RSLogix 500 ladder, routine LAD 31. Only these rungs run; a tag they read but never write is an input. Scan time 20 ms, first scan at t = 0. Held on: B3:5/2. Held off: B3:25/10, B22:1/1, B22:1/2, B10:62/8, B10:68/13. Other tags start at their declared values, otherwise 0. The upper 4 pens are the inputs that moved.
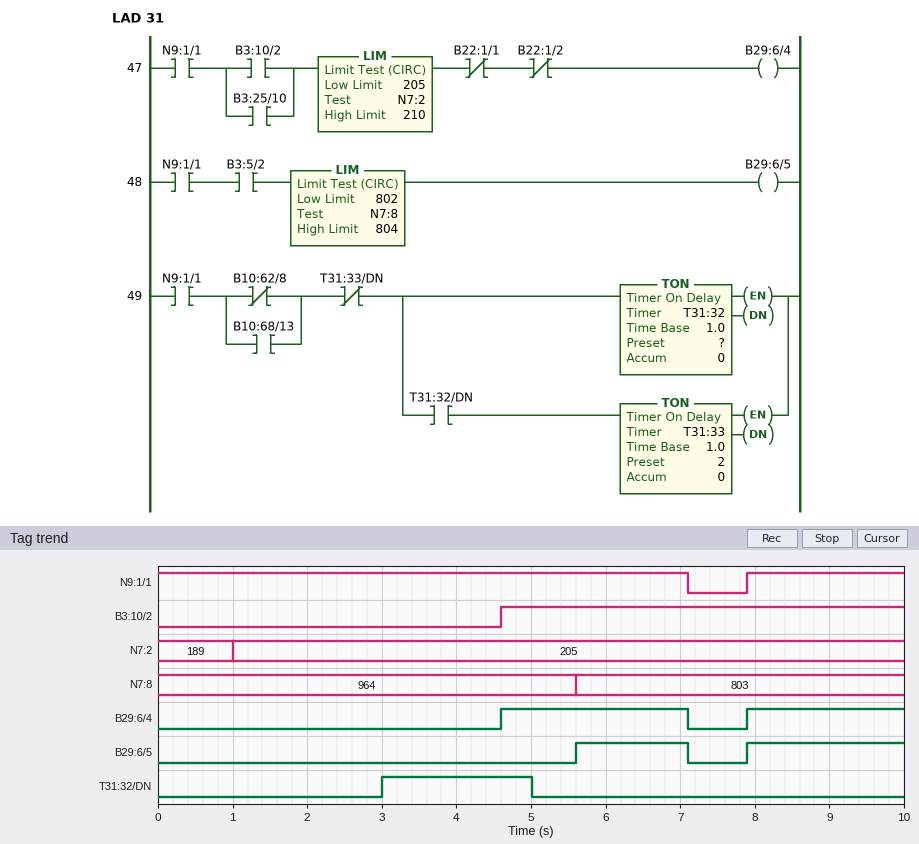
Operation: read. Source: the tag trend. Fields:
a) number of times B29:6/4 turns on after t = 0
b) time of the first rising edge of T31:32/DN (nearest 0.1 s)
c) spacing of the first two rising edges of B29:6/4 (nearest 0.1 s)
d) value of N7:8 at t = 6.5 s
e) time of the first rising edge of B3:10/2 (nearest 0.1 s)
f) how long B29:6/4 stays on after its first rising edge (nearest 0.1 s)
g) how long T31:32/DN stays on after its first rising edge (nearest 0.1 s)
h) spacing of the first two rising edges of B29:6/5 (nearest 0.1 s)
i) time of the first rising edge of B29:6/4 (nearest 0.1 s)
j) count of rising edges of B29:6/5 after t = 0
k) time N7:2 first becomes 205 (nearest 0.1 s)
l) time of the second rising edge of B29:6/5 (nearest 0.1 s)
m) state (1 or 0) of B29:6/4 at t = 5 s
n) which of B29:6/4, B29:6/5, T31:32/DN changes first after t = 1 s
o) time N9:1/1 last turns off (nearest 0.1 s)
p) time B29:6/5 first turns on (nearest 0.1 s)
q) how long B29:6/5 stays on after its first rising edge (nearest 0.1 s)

2
3.0 s
3.3 s
803
4.6 s
2.5 s
2.0 s
2.3 s
4.6 s
2
1.0 s
7.9 s
1
T31:32/DN
7.1 s
5.6 s
1.5 s
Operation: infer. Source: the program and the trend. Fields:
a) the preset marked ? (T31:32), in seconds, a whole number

3 s
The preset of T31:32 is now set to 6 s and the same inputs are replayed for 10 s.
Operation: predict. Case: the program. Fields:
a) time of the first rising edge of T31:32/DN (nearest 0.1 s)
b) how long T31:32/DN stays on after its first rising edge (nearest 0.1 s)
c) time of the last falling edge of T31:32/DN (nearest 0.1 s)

6.0 s
1.1 s
7.1 s
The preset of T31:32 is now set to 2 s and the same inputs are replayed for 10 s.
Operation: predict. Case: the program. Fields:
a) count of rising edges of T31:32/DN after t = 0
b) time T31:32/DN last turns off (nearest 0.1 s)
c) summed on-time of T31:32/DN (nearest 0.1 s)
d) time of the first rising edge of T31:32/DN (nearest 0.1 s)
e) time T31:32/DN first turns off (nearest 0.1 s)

3
7.1 s
3.2 s
2.0 s
4.0 s
